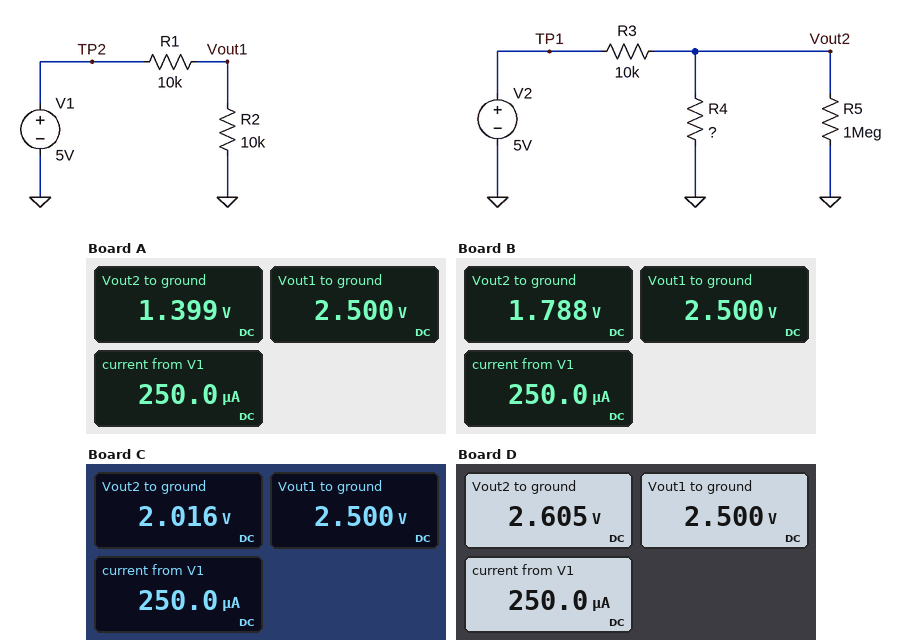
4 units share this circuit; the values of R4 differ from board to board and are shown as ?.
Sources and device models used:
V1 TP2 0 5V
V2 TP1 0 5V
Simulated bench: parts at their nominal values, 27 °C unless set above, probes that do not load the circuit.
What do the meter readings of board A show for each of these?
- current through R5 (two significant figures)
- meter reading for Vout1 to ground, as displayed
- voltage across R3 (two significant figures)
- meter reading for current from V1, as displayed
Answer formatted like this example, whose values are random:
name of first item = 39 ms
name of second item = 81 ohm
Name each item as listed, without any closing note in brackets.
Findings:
current through R5 = 1.4 µA
meter reading for Vout1 to ground, as displayed = 2.500 V
voltage across R3 = 3.6 V
meter reading for current from V1, as displayed = 250.0 µA
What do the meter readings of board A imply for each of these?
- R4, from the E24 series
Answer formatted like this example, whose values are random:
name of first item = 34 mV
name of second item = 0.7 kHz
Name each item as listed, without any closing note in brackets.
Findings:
R4, from the E24 series = 3.9 kΩ
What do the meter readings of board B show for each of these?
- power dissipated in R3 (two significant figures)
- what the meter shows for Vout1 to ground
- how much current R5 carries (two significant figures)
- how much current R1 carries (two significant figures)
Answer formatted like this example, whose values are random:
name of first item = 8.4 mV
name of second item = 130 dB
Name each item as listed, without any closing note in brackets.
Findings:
power dissipated in R3 = 1.0 mW
what the meter shows for Vout1 to ground = 2.500 V
how much current R5 carries = 1.8 µA
how much current R1 carries = 250 µA
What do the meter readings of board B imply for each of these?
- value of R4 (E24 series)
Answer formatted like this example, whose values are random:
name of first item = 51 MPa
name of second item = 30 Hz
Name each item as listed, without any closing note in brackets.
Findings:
value of R4 = 5.6 kΩ
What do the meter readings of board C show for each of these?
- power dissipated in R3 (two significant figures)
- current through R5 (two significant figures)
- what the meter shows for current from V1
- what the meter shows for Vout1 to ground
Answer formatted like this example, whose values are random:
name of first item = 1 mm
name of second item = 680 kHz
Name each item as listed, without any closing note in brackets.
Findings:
power dissipated in R3 = 890 µW
current through R5 = 2.0 µA
what the meter shows for current from V1 = 250.0 µA
what the meter shows for Vout1 to ground = 2.500 V
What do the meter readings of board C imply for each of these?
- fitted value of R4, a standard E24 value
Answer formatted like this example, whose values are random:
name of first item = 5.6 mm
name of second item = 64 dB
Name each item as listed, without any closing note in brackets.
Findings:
fitted value of R4, a standard E24 value = 6.8 kΩ
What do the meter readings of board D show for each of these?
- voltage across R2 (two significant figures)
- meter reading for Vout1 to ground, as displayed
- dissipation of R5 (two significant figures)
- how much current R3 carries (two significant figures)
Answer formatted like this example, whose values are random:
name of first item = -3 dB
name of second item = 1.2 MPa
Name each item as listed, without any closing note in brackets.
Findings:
voltage across R2 = 2.5 V
meter reading for Vout1 to ground, as displayed = 2.500 V
dissipation of R5 = 6.8 µW
how much current R3 carries = 240 µA
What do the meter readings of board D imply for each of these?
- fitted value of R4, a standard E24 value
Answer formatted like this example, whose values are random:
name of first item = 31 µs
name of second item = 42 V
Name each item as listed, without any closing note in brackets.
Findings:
fitted value of R4, a standard E24 value = 11 kΩ
